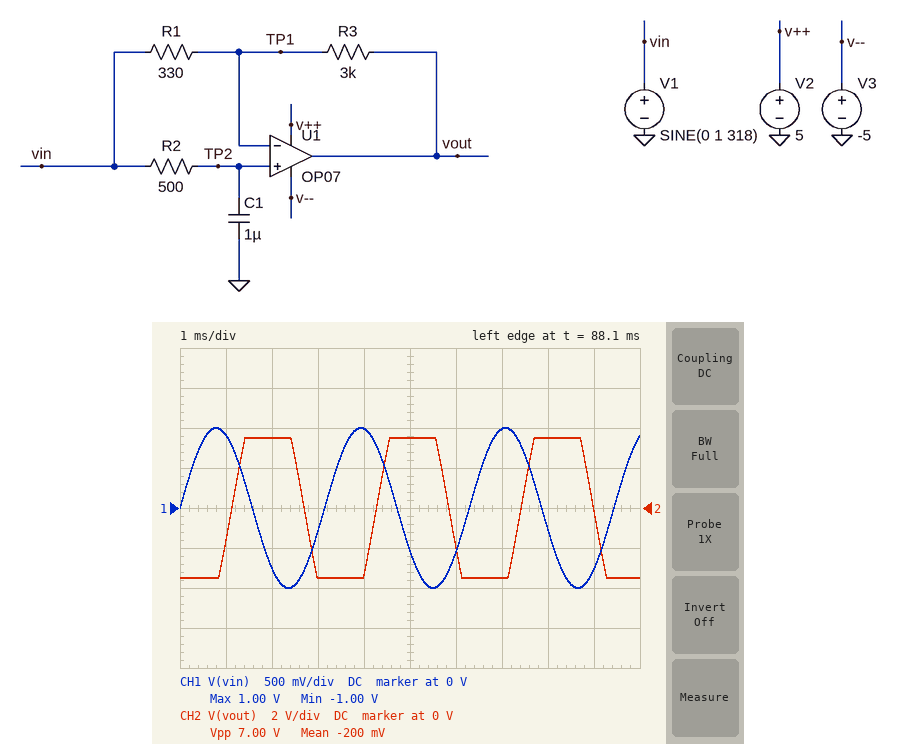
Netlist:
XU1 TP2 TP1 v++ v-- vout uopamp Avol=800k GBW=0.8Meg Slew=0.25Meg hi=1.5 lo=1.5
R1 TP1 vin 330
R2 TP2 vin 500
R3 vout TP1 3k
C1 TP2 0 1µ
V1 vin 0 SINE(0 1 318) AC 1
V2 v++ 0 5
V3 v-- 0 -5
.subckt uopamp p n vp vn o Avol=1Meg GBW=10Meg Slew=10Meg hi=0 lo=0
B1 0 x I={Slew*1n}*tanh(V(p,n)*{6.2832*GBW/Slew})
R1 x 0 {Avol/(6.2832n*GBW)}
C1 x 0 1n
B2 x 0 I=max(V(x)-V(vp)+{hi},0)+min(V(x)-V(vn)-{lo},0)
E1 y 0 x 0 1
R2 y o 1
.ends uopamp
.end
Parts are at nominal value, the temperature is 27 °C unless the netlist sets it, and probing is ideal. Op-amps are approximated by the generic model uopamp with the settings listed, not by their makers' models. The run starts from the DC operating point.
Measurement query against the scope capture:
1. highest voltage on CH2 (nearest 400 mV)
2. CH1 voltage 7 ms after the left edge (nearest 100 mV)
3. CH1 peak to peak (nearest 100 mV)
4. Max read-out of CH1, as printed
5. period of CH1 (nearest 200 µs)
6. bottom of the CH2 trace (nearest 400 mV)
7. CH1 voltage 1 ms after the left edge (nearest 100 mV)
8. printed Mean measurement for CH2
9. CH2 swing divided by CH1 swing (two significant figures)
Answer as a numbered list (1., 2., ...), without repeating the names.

1. 3.6 V
2. 1.0 V
3. 2.0 V
4. 1.00 V
5. 3.2 ms
6. -3.6 V
7. 900 mV
8. -200 mV
9. 3.5
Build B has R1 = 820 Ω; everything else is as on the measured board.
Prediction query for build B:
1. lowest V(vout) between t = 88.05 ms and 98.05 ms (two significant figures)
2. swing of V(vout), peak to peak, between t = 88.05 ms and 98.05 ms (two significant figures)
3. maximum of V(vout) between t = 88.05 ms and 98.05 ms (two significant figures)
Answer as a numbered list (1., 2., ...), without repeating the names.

1. -2.7 V
2. 5.4 V
3. 2.7 V
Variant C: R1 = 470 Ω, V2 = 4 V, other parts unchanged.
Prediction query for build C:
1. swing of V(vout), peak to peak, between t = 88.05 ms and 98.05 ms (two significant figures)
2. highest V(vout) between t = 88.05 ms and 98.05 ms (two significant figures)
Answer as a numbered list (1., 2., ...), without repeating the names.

1. 6.0 V
2. 2.5 V
